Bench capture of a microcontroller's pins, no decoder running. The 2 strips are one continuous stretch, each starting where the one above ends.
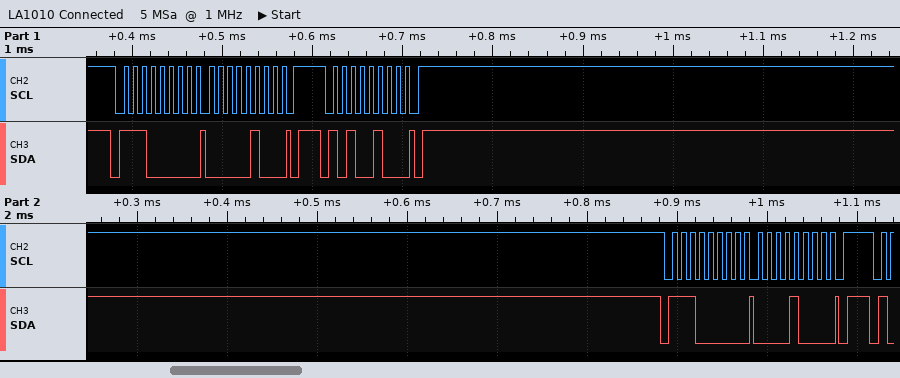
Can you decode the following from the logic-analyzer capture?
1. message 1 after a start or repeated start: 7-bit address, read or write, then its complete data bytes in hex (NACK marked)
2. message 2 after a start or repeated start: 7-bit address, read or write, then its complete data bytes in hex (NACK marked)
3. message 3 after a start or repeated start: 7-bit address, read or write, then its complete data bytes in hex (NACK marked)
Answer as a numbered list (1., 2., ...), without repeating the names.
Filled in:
1. 0x70 write: 04
2. 0x52 write
3. 0x70 write: 08
